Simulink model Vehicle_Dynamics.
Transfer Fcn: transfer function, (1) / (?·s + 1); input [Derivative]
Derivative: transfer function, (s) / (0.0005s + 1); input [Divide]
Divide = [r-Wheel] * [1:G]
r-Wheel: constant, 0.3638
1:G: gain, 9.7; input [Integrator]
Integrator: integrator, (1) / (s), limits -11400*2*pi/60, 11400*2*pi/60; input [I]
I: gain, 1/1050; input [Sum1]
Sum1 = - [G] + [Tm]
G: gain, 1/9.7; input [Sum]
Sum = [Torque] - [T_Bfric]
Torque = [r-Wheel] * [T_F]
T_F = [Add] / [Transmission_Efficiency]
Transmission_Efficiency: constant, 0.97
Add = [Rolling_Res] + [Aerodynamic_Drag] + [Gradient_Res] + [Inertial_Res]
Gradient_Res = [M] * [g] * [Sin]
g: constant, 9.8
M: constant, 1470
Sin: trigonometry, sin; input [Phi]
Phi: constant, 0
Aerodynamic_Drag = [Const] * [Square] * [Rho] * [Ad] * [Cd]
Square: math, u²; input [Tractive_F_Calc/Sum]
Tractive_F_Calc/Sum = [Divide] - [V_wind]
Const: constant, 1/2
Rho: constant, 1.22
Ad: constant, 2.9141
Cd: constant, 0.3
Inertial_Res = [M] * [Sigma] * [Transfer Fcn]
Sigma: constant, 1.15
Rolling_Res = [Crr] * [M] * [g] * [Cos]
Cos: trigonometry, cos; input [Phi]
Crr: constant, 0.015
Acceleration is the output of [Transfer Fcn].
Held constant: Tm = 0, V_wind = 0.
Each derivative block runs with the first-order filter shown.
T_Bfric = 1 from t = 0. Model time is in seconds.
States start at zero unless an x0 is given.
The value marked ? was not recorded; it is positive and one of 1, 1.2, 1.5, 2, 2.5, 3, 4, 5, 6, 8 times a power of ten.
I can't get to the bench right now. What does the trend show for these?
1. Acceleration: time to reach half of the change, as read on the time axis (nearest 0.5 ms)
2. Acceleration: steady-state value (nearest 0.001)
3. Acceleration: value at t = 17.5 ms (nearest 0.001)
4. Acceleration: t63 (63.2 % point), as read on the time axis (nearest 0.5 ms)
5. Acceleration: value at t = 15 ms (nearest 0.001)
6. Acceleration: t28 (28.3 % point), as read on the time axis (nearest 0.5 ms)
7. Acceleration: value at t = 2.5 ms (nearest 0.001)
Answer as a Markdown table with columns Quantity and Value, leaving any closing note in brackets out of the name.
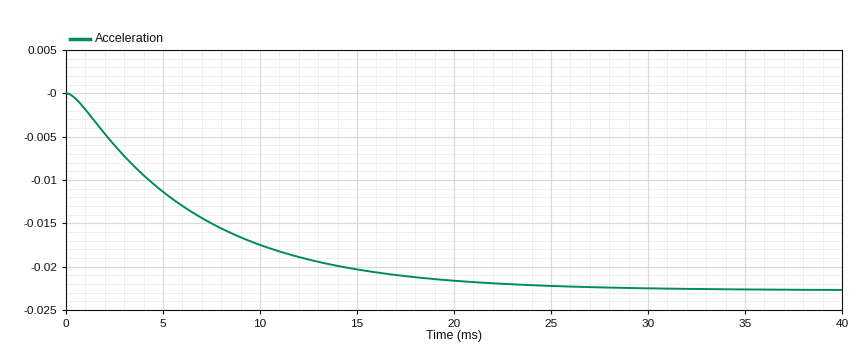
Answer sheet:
| Quantity | Value |
|---|---|
| Acceleration: time to reach half of the change, as read on the time axis | 5.0 ms |
| Acceleration: steady-state value | -0.023 |
| Acceleration: value at t = 17.5 ms | -0.021 |
| Acceleration: t63 (63.2 % point), as read on the time axis | 7.0 ms |
| Acceleration: value at t = 15 ms | -0.020 |
| Acceleration: t28 (28.3 % point), as read on the time axis | 2.5 ms |
| Acceleration: value at t = 2.5 ms | -0.006 |
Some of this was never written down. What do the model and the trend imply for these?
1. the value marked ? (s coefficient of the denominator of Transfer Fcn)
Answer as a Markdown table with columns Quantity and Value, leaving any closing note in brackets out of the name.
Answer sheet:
| Quantity | Value |
|---|---|
| the value marked ? | 0.008 |
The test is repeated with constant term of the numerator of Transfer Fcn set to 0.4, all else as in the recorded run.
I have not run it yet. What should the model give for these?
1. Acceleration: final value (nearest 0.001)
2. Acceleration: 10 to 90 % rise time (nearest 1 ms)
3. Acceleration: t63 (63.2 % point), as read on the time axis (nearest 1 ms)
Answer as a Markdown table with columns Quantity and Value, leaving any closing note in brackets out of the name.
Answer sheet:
| Quantity | Value |
|---|---|
| Acceleration: final value | -0.010 |
| Acceleration: 10 to 90 % rise time | 16 ms |
| Acceleration: t63 (63.2 % point), as read on the time axis | 8 ms |
